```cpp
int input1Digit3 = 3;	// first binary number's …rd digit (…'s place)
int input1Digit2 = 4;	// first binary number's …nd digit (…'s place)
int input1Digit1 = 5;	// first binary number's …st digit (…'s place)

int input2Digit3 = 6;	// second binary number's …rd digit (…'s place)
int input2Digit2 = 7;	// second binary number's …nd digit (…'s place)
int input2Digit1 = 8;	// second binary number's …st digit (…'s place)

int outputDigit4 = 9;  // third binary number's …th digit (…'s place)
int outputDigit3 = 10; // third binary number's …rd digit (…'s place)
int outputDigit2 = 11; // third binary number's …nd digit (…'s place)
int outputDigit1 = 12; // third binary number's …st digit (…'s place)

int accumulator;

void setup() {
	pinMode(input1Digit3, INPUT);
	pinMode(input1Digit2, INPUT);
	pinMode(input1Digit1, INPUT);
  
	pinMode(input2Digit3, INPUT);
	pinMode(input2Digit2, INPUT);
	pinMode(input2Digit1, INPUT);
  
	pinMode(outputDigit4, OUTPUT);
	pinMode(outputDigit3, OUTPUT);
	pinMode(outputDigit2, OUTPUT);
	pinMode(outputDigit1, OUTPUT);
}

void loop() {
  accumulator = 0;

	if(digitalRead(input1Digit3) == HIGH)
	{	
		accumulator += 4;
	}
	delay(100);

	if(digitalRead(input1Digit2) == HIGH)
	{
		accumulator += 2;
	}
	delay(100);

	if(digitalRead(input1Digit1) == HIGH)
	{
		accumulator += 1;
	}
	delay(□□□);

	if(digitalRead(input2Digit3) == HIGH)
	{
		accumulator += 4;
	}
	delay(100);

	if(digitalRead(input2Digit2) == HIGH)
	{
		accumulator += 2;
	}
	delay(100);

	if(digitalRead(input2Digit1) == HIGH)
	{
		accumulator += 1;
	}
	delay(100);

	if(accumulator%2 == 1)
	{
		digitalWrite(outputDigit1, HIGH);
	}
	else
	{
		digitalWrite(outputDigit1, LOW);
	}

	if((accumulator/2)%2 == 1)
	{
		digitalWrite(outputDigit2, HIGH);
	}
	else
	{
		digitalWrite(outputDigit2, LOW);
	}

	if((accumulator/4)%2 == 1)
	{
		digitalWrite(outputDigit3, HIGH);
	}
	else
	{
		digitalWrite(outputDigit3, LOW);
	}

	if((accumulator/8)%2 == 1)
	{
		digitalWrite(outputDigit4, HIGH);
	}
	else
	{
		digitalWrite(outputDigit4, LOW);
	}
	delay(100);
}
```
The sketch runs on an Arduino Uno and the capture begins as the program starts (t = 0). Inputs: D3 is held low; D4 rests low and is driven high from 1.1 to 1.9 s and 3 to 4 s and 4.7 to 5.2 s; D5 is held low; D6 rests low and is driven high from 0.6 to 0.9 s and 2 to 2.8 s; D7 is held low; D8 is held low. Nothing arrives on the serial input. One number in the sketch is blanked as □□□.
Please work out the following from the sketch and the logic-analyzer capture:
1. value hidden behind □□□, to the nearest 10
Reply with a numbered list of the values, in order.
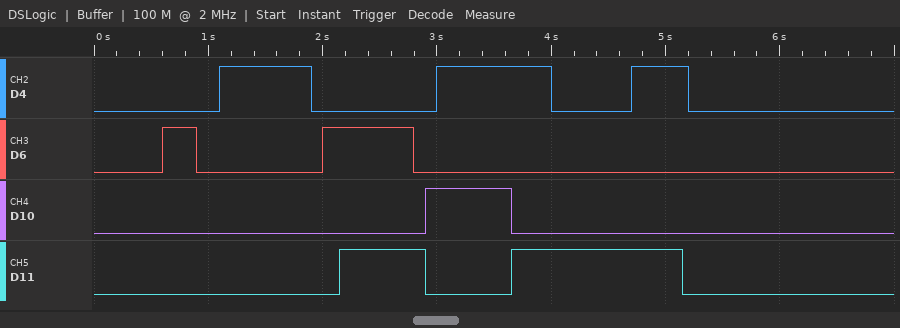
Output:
1. 150
